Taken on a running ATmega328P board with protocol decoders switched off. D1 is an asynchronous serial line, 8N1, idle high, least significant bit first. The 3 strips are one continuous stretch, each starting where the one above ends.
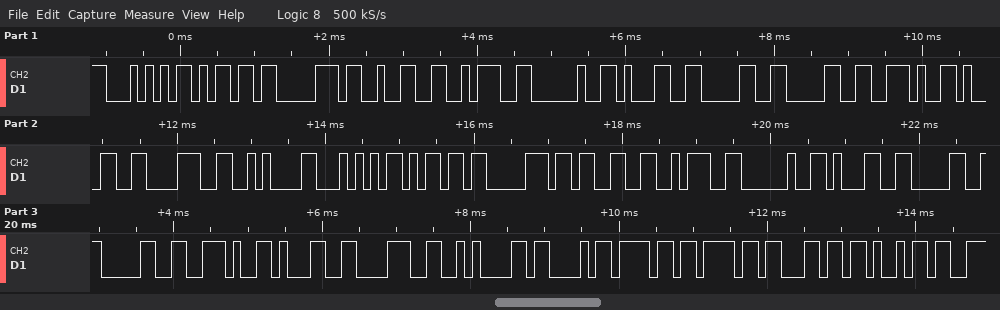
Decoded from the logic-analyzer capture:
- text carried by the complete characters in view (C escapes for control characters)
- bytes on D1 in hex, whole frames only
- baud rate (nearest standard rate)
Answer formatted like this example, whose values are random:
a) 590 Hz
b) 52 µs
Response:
a) "Tmp2: 100.18\nTmp3: 100.18\nCooli"
b) 54 6D 70 32 3A 20 31 30 30 2E 31 38 0A 54 6D 70 33 3A 20 31 30 30 2E 31 38 0A 43 6F 6F 6C 69
c) 9600 baud
